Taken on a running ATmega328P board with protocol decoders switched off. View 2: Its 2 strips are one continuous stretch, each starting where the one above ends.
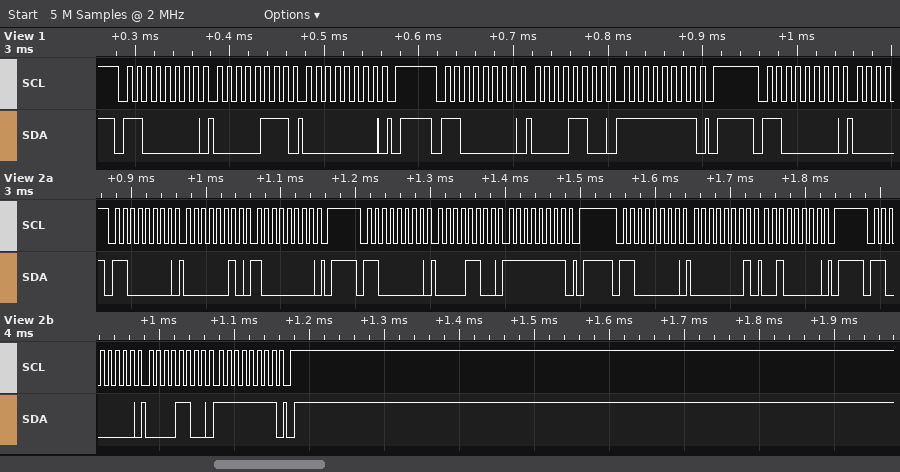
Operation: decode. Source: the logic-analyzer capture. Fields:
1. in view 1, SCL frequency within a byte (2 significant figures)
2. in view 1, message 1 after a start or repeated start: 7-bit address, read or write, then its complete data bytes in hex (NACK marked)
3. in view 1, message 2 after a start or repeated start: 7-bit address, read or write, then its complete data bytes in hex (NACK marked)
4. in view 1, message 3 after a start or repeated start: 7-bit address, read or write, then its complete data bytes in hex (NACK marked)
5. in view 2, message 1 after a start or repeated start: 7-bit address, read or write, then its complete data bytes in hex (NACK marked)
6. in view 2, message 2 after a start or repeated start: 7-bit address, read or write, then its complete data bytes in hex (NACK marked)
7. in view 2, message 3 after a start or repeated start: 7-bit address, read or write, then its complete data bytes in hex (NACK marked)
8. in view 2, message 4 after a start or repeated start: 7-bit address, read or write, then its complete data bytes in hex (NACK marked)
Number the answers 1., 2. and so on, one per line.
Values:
1. 100 kHz
2. 0x60 write: 07 00
3. 0x60 write: 0C FF
4. 0x60 write
5. 0x60 write: 02 80
6. 0x60 write: 0C FF
7. 0x60 write: 01 20
8. 0x60 write: 0C FF
